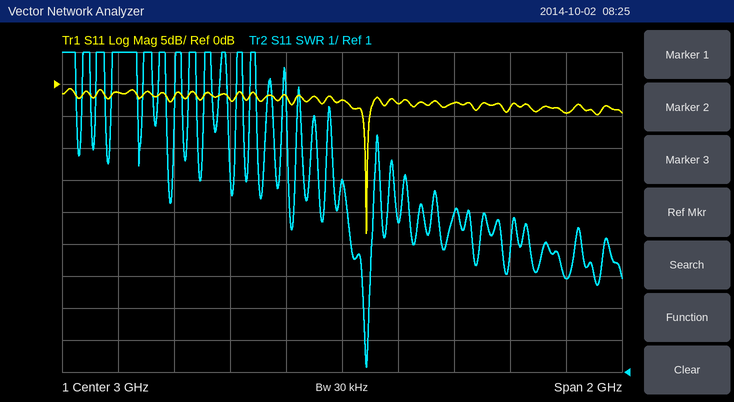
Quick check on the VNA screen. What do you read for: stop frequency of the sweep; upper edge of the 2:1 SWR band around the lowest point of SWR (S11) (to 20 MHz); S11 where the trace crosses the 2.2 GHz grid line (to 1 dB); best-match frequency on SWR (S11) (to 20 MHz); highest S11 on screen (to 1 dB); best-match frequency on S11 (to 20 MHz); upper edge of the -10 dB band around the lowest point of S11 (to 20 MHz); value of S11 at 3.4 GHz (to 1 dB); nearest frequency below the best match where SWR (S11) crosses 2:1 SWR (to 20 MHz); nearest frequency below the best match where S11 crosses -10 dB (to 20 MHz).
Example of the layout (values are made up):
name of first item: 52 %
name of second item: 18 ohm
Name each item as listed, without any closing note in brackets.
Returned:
stop frequency of the sweep: 4 GHz
upper edge of the 2:1 SWR band around the lowest point of SWR (S11): 3.10 GHz
S11 where the trace crosses the 2.2 GHz grid line: -1 dB
best-match frequency on SWR (S11): 3.08 GHz
highest S11 on screen: -1 dB
best-match frequency on S11: 3.08 GHz
upper edge of the -10 dB band around the lowest point of S11: 3.10 GHz
value of S11 at 3.4 GHz: -3 dB
nearest frequency below the best match where SWR (S11) crosses 2:1 SWR: 3.08 GHz
nearest frequency below the best match where S11 crosses -10 dB: 3.08 GHz
